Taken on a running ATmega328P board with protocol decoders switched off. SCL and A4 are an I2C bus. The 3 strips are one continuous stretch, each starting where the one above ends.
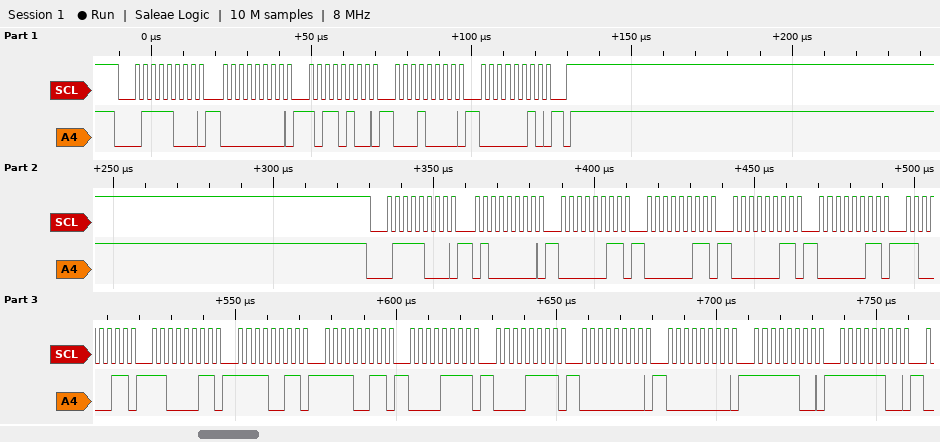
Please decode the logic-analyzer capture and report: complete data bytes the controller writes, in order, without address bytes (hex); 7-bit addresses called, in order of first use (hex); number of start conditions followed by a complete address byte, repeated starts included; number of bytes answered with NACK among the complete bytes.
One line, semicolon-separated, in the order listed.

00 B4 10 02 40 03 03 03 03 C3 C3 F3 F3 0F 0F 00 00 FC FC; 0x3C; 2; 0
